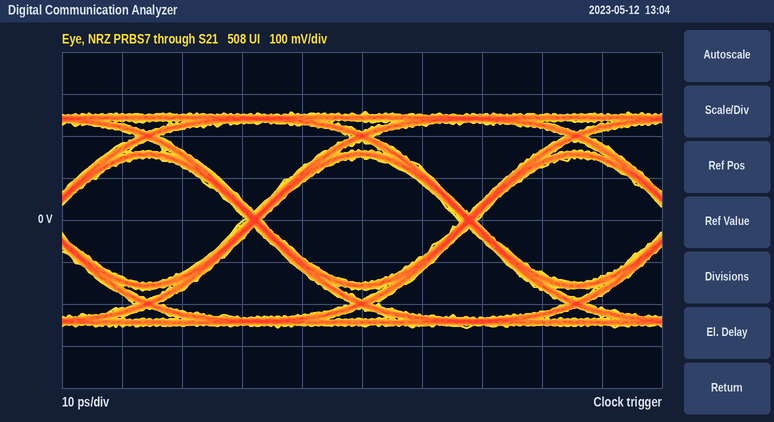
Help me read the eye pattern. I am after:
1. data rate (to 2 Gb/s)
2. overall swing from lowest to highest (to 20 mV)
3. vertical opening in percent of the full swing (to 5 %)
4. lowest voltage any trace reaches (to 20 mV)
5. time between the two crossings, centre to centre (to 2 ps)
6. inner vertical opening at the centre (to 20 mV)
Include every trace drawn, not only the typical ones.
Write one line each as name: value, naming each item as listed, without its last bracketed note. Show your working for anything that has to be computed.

data rate: 28 Gb/s
overall swing from lowest to highest: 520 mV
vertical opening in percent of the full swing: 300 mV / 520 mV ≈ 57.7 %, so 60 % to the nearest 5 %
lowest voltage any trace reaches: -260 mV
time between the two crossings, centre to centre: 36 ps
inner vertical opening at the centre: 300 mV
